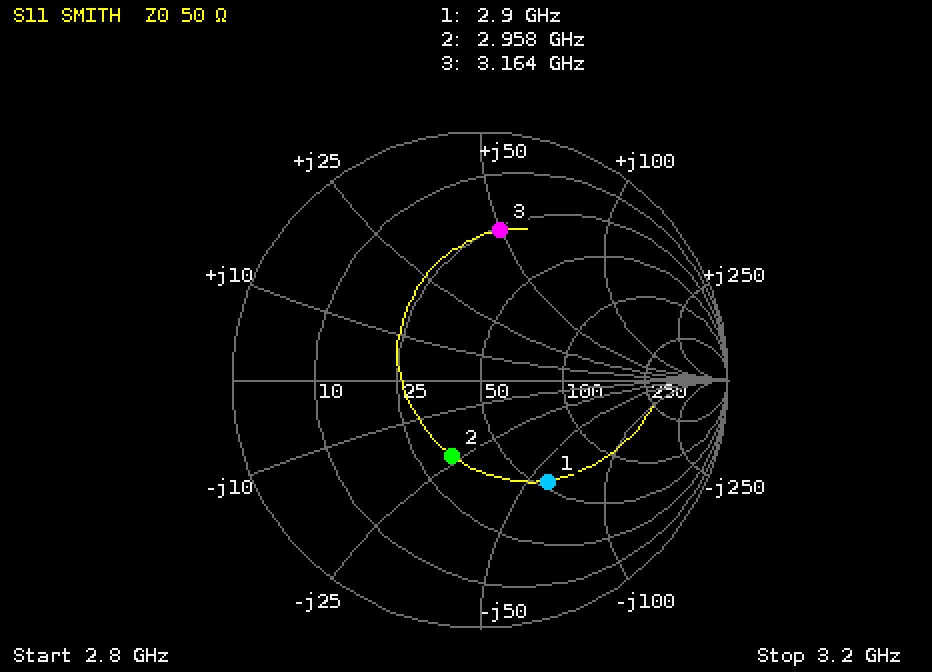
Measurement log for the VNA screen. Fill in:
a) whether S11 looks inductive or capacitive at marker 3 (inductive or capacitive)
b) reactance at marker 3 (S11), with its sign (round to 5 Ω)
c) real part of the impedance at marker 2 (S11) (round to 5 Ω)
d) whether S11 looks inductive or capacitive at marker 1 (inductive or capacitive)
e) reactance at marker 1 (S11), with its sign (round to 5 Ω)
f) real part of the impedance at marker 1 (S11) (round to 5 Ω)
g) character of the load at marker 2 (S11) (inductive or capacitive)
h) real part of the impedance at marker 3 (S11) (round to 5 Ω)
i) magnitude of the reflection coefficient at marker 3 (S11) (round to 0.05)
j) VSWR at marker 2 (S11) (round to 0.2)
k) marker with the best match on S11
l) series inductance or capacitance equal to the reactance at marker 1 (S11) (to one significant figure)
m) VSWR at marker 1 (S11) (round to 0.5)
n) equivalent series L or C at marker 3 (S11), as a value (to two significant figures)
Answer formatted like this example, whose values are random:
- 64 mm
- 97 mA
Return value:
- inductive
- +50 Ω
- 35 Ω
- capacitive
- -60 Ω
- 55 Ω
- capacitive
- 25 Ω
- 0.60
- 2.0
- marker 2
- 900 fF
- 3.0
- 2.5 nH
